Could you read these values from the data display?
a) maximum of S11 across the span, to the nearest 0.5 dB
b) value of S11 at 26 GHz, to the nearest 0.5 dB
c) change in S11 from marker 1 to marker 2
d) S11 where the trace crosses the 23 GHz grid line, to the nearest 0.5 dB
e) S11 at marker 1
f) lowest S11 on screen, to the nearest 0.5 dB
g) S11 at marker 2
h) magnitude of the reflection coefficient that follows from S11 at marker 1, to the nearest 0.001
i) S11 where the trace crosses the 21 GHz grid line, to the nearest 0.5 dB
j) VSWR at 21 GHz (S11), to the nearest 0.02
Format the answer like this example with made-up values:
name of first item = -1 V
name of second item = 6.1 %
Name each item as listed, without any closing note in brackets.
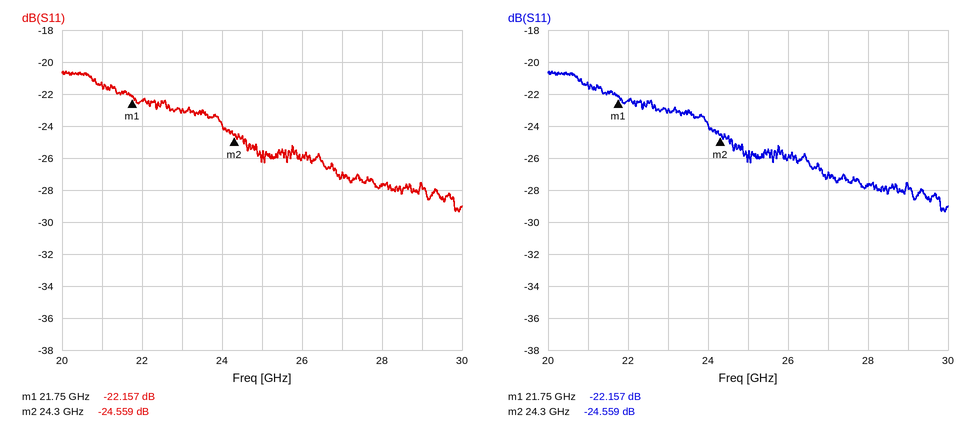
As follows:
maximum of S11 across the span, to the nearest 0.5 dB = -20.5 dB
value of S11 at 26 GHz, to the nearest 0.5 dB = -26.0 dB
change in S11 from marker 1 to marker 2 = -2.402 dB
S11 where the trace crosses the 23 GHz grid line, to the nearest 0.5 dB = -23.0 dB
S11 at marker 1 = -22.157 dB
lowest S11 on screen, to the nearest 0.5 dB = -29.5 dB
S11 at marker 2 = -24.559 dB
magnitude of the reflection coefficient that follows from S11 at marker 1, to the nearest 0.001 = 0.078
S11 where the trace crosses the 21 GHz grid line, to the nearest 0.5 dB = -21.5 dB
VSWR at 21 GHz (S11), to the nearest 0.02 = 1.18
